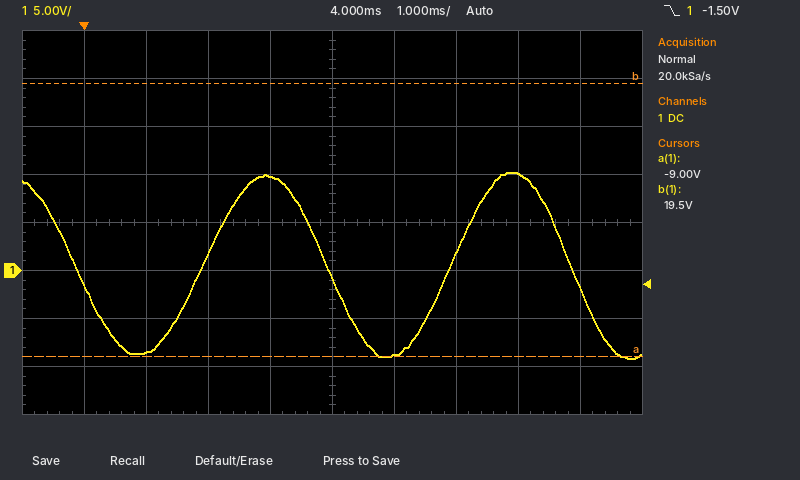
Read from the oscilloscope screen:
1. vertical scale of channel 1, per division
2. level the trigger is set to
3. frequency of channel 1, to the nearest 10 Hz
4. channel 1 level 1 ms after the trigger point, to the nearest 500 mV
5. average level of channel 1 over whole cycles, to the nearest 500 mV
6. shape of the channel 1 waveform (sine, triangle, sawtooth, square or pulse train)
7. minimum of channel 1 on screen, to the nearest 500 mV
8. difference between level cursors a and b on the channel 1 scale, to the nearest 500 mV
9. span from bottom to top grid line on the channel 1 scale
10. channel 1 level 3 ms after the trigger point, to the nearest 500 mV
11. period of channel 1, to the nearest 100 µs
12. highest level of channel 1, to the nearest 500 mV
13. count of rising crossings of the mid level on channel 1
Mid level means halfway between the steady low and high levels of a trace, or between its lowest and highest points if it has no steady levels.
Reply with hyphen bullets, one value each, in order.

- 5 V
- -1.50 V
- 250 Hz
- -8.5 V
- 500 mV
- sine
- -9.0 V
- 28.5 V
- 40 V
- 10.0 V
- 4.0 ms
- 10.0 V
- 2
